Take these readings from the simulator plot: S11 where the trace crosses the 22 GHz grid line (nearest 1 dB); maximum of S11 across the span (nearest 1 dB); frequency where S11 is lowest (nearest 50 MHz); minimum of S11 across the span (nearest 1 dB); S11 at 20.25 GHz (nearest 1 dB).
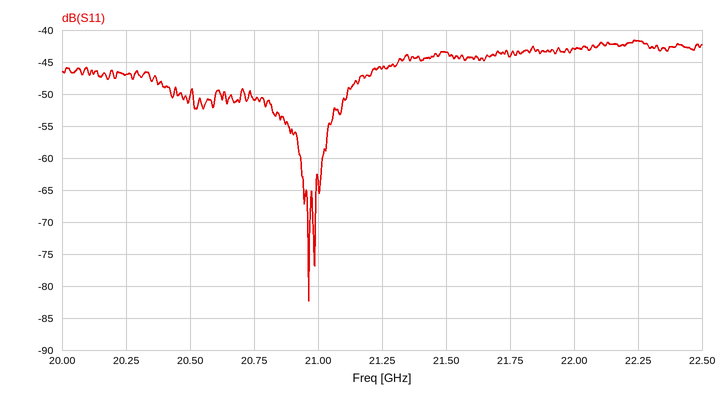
-43 dB
-42 dB
20.95 GHz
-82 dB
-47 dB
